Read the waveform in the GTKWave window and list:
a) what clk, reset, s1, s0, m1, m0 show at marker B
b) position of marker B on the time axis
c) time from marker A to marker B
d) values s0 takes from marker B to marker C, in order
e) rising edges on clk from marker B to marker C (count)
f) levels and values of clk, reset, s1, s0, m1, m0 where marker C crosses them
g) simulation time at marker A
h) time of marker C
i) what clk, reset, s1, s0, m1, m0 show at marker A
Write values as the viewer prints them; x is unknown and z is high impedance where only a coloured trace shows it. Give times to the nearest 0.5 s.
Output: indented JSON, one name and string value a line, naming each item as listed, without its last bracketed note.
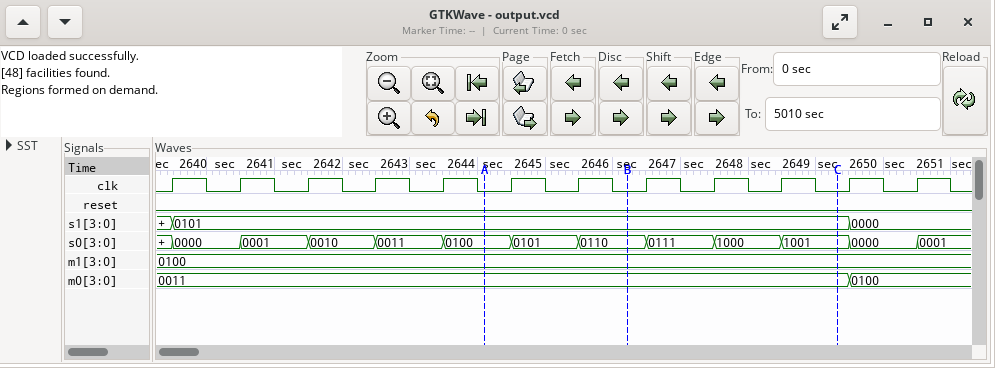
{
  "what clk, reset, s1, s0, m1, m0 show at marker B": "clk=0, reset=0, s1=0101, s0=0110, m1=0100, m0=0011",
  "position of marker B on the time axis": "2646 s",
  "time from marker A to marker B": "2 s",
  "values s0 takes from marker B to marker C, in order": "0110, 0111, 1000, 1001",
  "rising edges on clk from marker B to marker C": "3",
  "levels and values of clk, reset, s1, s0, m1, m0 where marker C crosses them": "clk=0, reset=0, s1=0101, s0=1001, m1=0100, m0=0011",
  "simulation time at marker A": "2644 s",
  "time of marker C": "2649.5 s",
  "what clk, reset, s1, s0, m1, m0 show at marker A": "clk=0, reset=0, s1=0101, s0=0100, m1=0100, m0=0011"
}
